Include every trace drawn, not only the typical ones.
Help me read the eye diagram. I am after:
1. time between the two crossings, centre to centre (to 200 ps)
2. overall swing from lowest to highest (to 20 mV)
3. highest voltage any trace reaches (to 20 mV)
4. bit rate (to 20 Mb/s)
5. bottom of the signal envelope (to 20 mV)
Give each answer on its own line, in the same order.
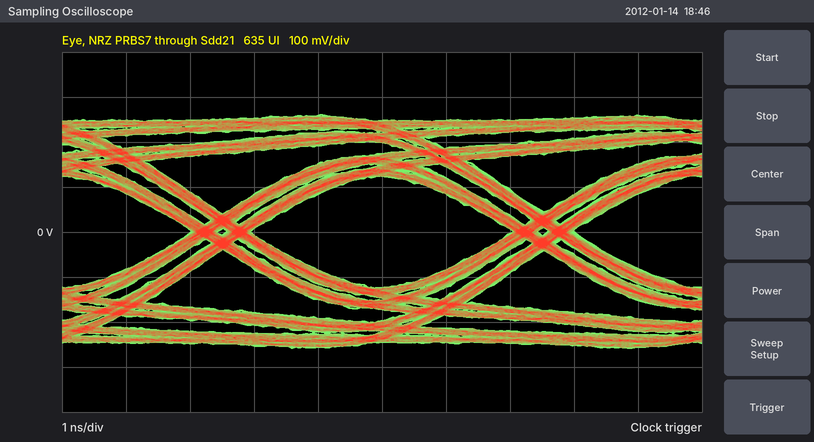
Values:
5.0 ns
520 mV
260 mV
200 Mb/s
-260 mV
